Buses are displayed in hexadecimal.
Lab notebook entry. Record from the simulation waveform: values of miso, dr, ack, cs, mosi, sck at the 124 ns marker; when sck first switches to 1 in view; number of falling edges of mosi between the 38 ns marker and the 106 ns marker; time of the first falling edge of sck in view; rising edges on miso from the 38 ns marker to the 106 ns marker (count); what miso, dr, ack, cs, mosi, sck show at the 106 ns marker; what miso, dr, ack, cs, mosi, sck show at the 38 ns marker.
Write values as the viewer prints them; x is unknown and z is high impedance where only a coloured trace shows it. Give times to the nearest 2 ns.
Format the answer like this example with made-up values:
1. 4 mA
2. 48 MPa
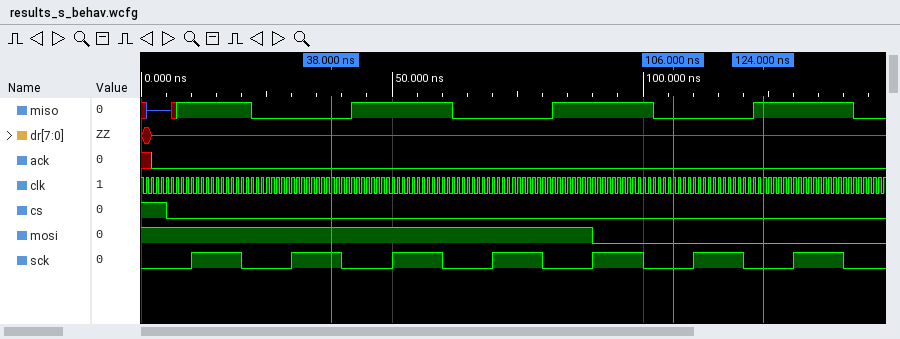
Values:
1. miso=1, dr=z, ack=0, cs=0, mosi=0, sck=0
2. 10 ns
3. 1
4. 20 ns
5. 2
6. miso=0, dr=z, ack=0, cs=0, mosi=0, sck=0
7. miso=0, dr=z, ack=0, cs=0, mosi=1, sck=1
